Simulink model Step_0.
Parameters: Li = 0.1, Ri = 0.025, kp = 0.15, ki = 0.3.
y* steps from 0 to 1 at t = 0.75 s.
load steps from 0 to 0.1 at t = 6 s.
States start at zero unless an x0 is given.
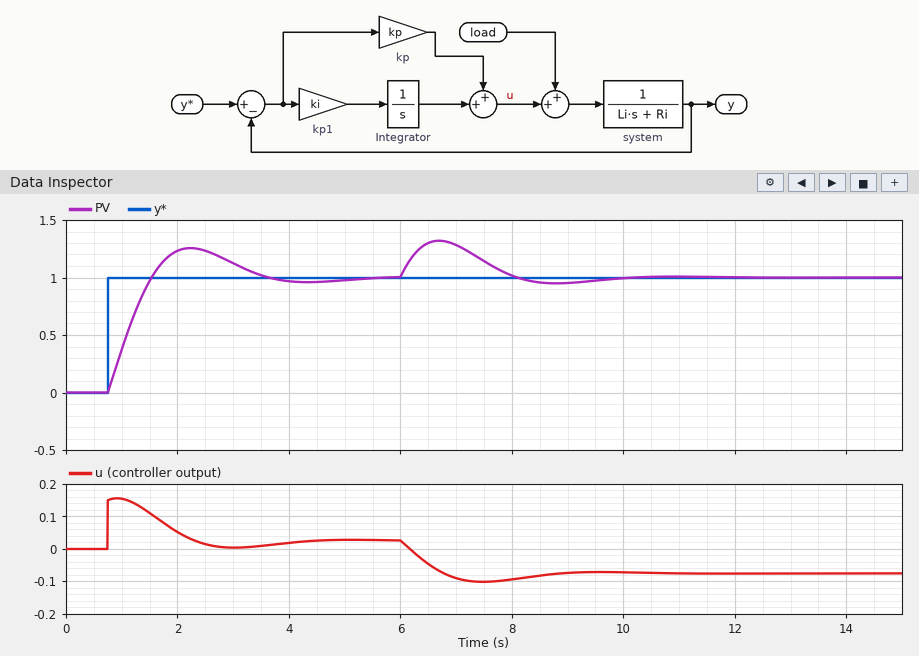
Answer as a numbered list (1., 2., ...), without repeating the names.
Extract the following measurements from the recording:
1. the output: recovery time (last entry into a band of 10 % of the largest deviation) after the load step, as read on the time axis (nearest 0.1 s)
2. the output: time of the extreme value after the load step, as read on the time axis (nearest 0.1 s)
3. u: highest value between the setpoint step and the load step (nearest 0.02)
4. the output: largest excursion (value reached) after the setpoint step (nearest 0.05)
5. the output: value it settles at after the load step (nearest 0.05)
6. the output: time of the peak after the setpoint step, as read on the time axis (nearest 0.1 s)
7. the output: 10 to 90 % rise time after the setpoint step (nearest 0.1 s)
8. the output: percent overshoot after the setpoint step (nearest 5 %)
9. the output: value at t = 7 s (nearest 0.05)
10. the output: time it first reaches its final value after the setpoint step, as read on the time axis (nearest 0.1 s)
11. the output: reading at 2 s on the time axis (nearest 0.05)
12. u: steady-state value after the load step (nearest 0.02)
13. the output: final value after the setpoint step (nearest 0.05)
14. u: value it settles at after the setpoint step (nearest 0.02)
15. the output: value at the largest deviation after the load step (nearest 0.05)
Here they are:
1. 9.4 s
2. 6.7 s
3. 0.16
4. 1.25
5. 1.00
6. 2.2 s
7. 0.6 s
8. 25 %
9. 1.30
10. 1.5 s
11. 1.25
12. -0.08
13. 1.00
14. 0.02
15. 1.30
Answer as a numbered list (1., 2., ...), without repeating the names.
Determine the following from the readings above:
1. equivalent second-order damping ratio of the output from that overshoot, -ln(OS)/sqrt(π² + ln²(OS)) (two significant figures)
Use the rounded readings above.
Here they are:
1. 0.40
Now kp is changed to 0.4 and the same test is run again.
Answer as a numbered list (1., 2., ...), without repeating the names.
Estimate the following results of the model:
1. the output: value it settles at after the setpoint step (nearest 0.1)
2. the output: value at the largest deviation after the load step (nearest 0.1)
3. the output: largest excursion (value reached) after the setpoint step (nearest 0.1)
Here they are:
1. 1.0
2. 1.2
3. 1.1
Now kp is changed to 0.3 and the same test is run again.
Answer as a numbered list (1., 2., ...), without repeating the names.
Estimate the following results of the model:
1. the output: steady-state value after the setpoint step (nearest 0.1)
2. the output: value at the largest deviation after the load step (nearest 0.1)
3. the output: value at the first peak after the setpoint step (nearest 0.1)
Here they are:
1. 1.0
2. 1.2
3. 1.1
